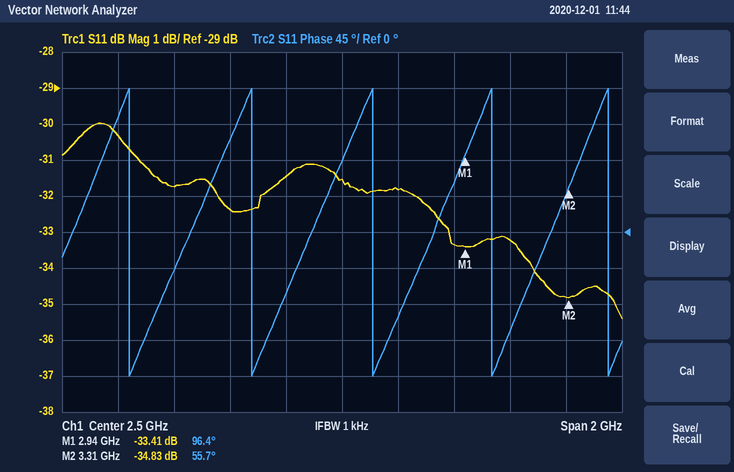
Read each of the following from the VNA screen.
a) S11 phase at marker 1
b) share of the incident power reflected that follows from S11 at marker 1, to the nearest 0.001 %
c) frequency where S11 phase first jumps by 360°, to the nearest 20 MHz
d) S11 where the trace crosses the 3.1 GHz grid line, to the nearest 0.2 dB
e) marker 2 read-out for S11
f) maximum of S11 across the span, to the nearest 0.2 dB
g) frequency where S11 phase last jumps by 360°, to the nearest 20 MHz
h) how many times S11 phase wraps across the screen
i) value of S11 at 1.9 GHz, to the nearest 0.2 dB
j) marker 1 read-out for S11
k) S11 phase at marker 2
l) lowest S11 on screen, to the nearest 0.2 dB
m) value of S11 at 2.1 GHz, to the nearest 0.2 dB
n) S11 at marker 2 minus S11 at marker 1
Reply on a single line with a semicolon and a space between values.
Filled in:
96.4°; 0.046 %; 1.74 GHz; -33.2 dB; -34.83 dB; -30.0 dB; 3.46 GHz; 5; -31.8 dB; -33.41 dB; 55.7°; -35.4 dB; -32.4 dB; -1.42 dB
